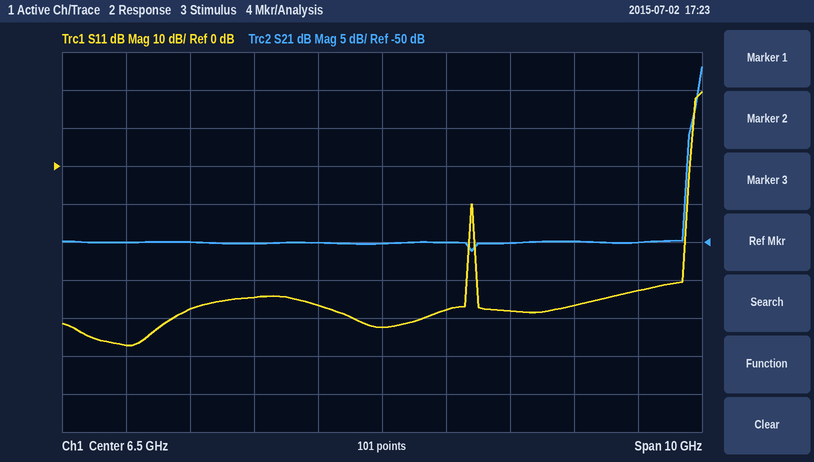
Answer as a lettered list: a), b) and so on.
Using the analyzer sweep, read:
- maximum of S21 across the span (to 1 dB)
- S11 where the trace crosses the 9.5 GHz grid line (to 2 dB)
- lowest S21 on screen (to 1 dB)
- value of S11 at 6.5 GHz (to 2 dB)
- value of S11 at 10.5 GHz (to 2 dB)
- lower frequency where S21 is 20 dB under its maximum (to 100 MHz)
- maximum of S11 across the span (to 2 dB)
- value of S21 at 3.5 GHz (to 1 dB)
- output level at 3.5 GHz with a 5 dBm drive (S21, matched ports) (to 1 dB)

a) -27 dB
b) -36 dB
c) -51 dB
d) -42 dB
e) -32 dB
f) 11.2 GHz
g) 20 dB
h) -50 dB
i) -45 dBm
